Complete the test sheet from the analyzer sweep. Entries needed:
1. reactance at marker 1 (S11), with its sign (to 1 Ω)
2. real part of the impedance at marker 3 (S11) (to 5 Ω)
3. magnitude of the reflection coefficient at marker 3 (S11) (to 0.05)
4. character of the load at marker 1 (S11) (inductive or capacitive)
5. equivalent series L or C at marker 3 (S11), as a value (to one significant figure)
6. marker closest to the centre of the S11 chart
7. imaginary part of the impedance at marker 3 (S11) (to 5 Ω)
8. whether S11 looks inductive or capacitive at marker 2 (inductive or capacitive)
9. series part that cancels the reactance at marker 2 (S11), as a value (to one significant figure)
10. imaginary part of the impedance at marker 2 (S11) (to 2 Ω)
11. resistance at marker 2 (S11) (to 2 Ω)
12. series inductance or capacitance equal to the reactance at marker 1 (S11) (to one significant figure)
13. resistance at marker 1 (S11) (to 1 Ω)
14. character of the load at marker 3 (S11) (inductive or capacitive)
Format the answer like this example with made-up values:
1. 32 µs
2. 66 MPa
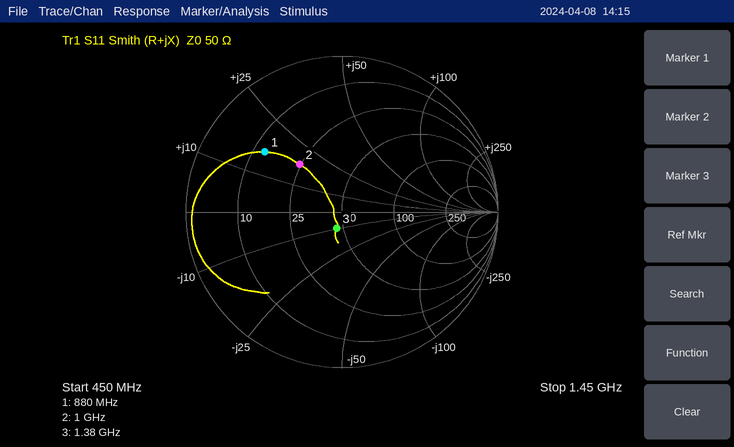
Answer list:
1. +16 Ω
2. 45 Ω
3. 0.10
4. inductive
5. 10 pF
6. marker 3
7. -10 Ω
8. inductive
9. 9 pF
10. +18 Ω
11. 24 Ω
12. 3 nH
13. 13 Ω
14. capacitive
